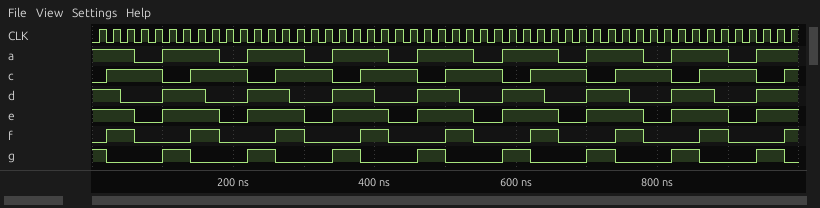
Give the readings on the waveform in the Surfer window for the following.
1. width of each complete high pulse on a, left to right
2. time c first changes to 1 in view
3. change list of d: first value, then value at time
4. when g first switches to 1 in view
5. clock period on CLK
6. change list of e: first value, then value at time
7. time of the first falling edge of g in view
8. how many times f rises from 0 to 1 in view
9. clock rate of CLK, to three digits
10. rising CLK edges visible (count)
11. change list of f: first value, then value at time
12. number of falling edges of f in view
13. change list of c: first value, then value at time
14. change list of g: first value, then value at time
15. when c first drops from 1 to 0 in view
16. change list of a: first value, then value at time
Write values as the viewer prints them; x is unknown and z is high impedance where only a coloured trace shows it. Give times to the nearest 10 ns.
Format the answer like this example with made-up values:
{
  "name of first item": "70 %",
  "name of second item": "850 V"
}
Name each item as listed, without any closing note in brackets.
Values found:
{
  "width of each complete high pulse on a, left to right": "80 ns, 80 ns, 80 ns, 80 ns, 80 ns, 80 ns, 80 ns",
  "time c first changes to 1 in view": "20 ns",
  "change list of d: first value, then value at time": "1, 0 at 40 ns, 1 at 100 ns, 0 at 160 ns, 1 at 220 ns, 0 at 280 ns, 1 at 340 ns, 0 at 400 ns, 1 at 460 ns, 0 at 520 ns, 1 at 580 ns, 0 at 640 ns, 1 at 700 ns, 0 at 760 ns, 1 at 820 ns, 0 at 880 ns, 1 at 940 ns",
  "when g first switches to 1 in view": "100 ns",
  "clock period on CLK": "20 ns",
  "change list of e: first value, then value at time": "1, 0 at 60 ns, 1 at 100 ns, 0 at 180 ns, 1 at 220 ns, 0 at 300 ns, 1 at 340 ns, 0 at 420 ns, 1 at 460 ns, 0 at 540 ns, 1 at 580 ns, 0 at 660 ns, 1 at 700 ns, 0 at 780 ns, 1 at 820 ns, 0 at 900 ns, 1 at 940 ns",
  "time of the first falling edge of g in view": "20 ns",
  "how many times f rises from 0 to 1 in view": "9",
  "clock rate of CLK, to three digits": "50.0 MHz",
  "rising CLK edges visible": "50",
  "change list of f: first value, then value at time": "0, 1 at 20 ns, 0 at 60 ns, 1 at 140 ns, 0 at 180 ns, 1 at 260 ns, 0 at 300 ns, 1 at 380 ns, 0 at 420 ns, 1 at 500 ns, 0 at 540 ns, 1 at 620 ns, 0 at 660 ns, 1 at 740 ns, 0 at 780 ns, 1 at 860 ns, 0 at 900 ns, 1 at 980 ns",
  "number of falling edges of f in view": "8",
  "change list of c: first value, then value at time": "0, 1 at 20 ns, 0 at 100 ns, 1 at 140 ns, 0 at 220 ns, 1 at 260 ns, 0 at 340 ns, 1 at 380 ns, 0 at 460 ns, 1 at 500 ns, 0 at 580 ns, 1 at 620 ns, 0 at 700 ns, 1 at 740 ns, 0 at 820 ns, 1 at 860 ns, 0 at 940 ns, 1 at 980 ns",
  "change list of g: first value, then value at time": "1, 0 at 20 ns, 1 at 100 ns, 0 at 140 ns, 1 at 220 ns, 0 at 260 ns, 1 at 340 ns, 0 at 380 ns, 1 at 460 ns, 0 at 500 ns, 1 at 580 ns, 0 at 620 ns, 1 at 700 ns, 0 at 740 ns, 1 at 820 ns, 0 at 860 ns, 1 at 940 ns, 0 at 980 ns",
  "when c first drops from 1 to 0 in view": "100 ns",
  "change list of a: first value, then value at time": "1, 0 at 60 ns, 1 at 100 ns, 0 at 180 ns, 1 at 220 ns, 0 at 300 ns, 1 at 340 ns, 0 at 420 ns, 1 at 460 ns, 0 at 540 ns, 1 at 580 ns, 0 at 660 ns, 1 at 700 ns, 0 at 780 ns, 1 at 820 ns, 0 at 900 ns, 1 at 940 ns"
}
